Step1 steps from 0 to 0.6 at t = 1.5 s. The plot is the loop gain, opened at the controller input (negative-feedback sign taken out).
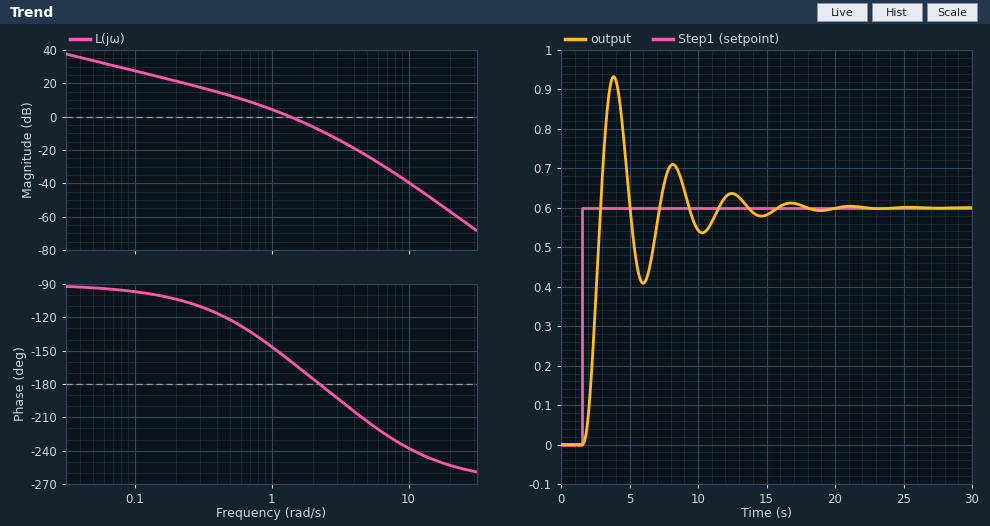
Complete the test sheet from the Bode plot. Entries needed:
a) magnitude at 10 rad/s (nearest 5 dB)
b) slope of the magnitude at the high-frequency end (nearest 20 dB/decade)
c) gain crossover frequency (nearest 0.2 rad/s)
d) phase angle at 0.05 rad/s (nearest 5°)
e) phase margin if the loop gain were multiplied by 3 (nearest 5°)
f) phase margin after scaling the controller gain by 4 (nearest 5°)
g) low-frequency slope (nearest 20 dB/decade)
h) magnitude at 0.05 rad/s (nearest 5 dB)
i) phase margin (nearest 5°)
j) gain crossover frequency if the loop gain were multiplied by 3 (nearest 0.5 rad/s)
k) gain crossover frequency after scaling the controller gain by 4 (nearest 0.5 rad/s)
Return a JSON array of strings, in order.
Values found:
["-40 dB", "-60 dB/decade", "1.4 rad/s", "-95°", "-5°", "-10°", "-20 dB/decade", "35 dB", "20°", "2.5 rad/s", "3.0 rad/s"]
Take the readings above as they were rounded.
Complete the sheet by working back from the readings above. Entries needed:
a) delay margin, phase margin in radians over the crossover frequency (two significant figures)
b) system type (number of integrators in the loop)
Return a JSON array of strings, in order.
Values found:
["0.25 s", "1"]
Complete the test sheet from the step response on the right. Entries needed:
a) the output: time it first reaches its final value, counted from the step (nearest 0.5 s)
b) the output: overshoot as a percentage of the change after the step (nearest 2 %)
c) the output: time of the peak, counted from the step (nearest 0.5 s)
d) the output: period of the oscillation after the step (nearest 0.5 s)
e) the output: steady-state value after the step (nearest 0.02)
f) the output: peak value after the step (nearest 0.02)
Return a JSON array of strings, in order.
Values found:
["1.5 s", "56 %", "2.5 s", "4.5 s", "0.60", "0.94"]
